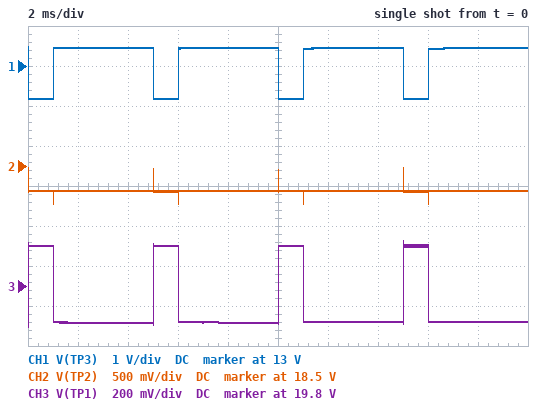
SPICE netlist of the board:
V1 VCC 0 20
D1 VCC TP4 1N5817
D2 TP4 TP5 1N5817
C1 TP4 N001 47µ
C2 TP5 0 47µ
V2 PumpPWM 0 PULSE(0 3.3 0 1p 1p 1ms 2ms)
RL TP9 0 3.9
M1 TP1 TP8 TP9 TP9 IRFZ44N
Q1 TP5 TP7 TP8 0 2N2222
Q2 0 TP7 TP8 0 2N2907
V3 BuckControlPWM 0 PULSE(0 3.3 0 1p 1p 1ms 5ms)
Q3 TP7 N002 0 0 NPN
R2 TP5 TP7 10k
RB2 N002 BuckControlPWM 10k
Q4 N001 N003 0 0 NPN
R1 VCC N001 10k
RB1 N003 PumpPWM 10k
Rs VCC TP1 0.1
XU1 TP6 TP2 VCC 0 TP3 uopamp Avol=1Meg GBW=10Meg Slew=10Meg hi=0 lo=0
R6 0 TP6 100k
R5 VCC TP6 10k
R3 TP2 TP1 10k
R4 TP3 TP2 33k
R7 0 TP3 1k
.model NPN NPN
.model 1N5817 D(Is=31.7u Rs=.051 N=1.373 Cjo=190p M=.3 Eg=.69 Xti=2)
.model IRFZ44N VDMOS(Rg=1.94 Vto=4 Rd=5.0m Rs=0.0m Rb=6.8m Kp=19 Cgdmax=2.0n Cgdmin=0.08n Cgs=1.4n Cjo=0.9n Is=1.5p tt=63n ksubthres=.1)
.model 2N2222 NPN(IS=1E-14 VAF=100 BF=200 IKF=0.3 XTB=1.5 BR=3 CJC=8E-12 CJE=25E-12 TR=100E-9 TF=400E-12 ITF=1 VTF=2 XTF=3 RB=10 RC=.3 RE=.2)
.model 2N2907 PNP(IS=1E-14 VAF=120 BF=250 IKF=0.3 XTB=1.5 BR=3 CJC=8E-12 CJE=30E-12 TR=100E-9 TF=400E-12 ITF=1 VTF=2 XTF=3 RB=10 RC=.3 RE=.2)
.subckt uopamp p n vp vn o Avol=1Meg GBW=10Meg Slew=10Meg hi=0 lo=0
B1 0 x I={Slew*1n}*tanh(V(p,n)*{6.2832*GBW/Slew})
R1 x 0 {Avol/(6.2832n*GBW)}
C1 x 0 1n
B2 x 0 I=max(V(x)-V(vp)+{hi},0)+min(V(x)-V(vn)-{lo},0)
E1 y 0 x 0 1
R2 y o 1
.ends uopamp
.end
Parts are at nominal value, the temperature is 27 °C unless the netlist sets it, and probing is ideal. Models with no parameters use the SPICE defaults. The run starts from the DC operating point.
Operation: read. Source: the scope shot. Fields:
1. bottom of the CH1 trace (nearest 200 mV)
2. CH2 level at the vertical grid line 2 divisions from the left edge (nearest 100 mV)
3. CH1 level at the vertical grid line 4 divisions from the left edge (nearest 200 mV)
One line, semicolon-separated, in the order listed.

12.2 V; 18.2 V; 13.4 V
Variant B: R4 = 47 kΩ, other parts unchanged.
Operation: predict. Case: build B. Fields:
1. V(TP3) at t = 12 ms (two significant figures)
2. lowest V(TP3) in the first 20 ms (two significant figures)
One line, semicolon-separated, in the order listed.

11 V; 9.6 V
